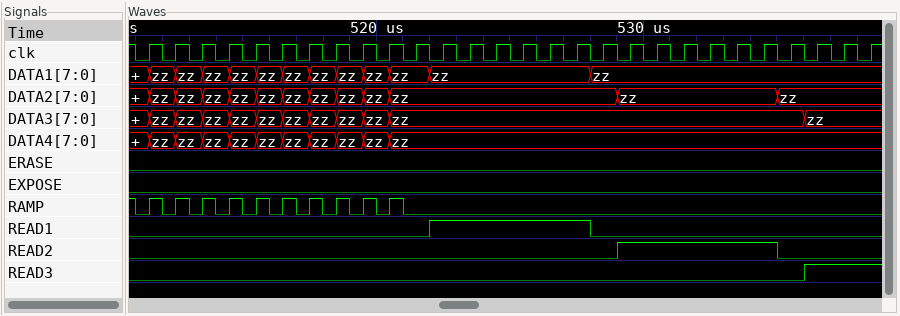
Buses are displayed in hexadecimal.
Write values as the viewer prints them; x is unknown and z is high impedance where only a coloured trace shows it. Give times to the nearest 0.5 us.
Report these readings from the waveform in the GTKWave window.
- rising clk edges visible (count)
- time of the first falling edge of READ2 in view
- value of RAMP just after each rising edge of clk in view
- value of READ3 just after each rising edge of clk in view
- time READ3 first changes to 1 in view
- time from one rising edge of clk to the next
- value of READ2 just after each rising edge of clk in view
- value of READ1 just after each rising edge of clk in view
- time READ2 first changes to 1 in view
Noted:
28
535 us
1 1 1 1 1 1 1 1 1 1 0 0 0 0 0 0 0 0 0 0 0 0 0 0 0 0 0 0
0 0 0 0 0 0 0 0 0 0 0 0 0 0 0 0 0 0 0 0 0 0 0 0 0 1 1 1
536 us
1 us
0 0 0 0 0 0 0 0 0 0 0 0 0 0 0 0 0 0 1 1 1 1 1 1 0 0 0 0
0 0 0 0 0 0 0 0 0 0 0 1 1 1 1 1 1 0 0 0 0 0 0 0 0 0 0 0
529 us
